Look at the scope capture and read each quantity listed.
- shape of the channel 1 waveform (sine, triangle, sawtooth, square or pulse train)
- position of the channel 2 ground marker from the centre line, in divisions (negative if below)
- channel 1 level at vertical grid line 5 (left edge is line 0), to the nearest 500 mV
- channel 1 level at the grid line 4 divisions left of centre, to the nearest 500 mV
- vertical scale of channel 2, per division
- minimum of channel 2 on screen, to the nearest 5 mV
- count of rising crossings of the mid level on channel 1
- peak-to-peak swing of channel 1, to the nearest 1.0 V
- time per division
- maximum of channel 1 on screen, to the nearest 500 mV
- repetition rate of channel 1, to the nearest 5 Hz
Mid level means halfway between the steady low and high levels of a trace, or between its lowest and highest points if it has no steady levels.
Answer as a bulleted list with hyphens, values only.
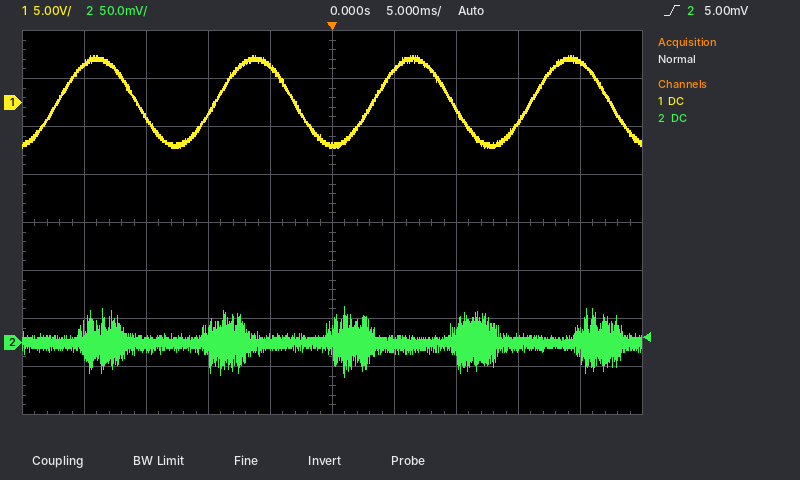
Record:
- sine
- -2.5 div
- -4.5 V
- 4.0 V
- 50 mV
- -35 mV
- 4
- 10.0 V
- 5 ms
- 5.0 V
- 80 Hz
